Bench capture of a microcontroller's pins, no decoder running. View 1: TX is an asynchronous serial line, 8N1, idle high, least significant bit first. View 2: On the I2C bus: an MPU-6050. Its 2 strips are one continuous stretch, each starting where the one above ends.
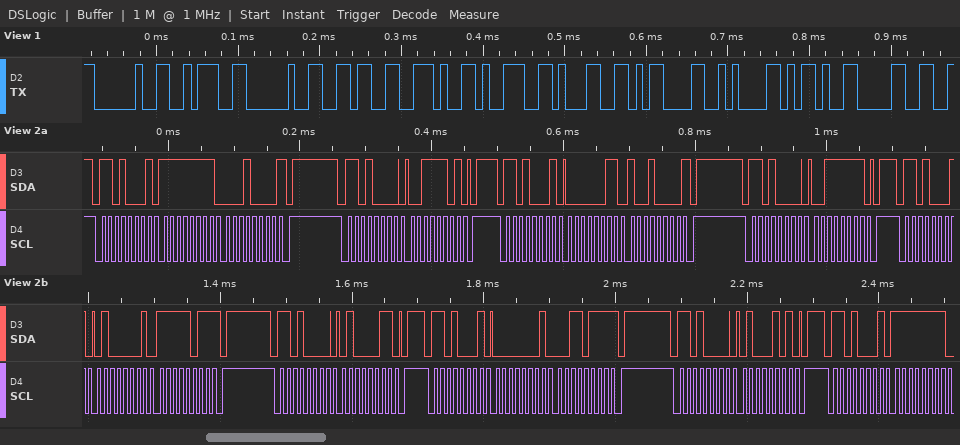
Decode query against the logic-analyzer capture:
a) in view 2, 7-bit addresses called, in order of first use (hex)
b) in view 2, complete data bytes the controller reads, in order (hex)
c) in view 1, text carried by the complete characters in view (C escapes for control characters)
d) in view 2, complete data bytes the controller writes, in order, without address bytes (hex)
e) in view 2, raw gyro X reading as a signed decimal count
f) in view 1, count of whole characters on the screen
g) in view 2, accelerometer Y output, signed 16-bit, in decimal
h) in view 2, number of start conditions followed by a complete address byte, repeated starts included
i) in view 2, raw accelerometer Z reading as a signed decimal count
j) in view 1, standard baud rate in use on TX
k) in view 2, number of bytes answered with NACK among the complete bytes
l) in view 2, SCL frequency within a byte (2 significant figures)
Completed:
0x68
FF 10 03 90 41 FB 01 37 FF
" : 6.91\r\n-0"
3D 3F 43 45
311
11
912
9
16891
115200 baud
4
100 kHz
